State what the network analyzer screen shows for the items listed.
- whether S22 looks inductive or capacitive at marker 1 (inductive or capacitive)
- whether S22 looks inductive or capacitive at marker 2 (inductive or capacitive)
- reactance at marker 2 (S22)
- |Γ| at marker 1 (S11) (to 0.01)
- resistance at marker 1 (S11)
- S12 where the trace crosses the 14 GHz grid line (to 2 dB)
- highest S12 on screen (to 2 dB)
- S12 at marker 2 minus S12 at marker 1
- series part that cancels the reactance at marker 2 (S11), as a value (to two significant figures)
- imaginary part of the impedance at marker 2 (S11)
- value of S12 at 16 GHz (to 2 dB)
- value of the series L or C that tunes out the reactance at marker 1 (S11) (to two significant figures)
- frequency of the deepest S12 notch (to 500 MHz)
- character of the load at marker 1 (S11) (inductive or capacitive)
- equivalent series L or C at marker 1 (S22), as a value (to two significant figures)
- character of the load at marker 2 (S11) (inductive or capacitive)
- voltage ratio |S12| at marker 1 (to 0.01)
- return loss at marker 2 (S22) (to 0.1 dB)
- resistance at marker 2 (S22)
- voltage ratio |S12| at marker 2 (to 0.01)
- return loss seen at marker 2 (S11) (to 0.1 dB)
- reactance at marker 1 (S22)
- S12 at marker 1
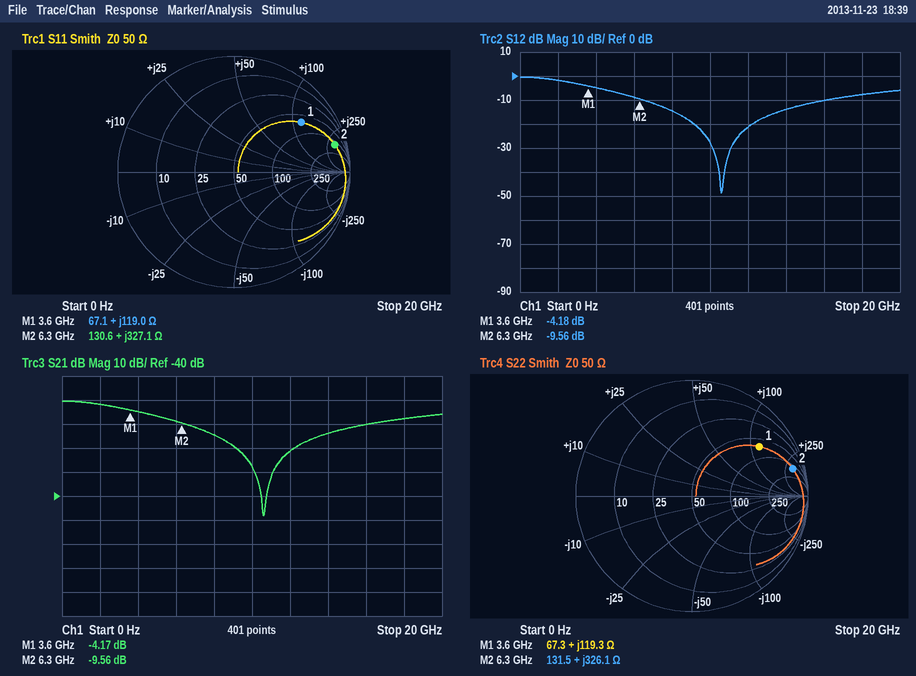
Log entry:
inductive
inductive
+326.1 Ω
0.72
67.1 Ω
-14 dB
0 dB
-5.38 dB
77 fF
+327.1 Ω
-10 dB
370 fF
10.5 GHz
inductive
5.3 nH
inductive
0.62
0.9 dB
131.5 Ω
0.33
0.9 dB
+119.3 Ω
-4.18 dB
